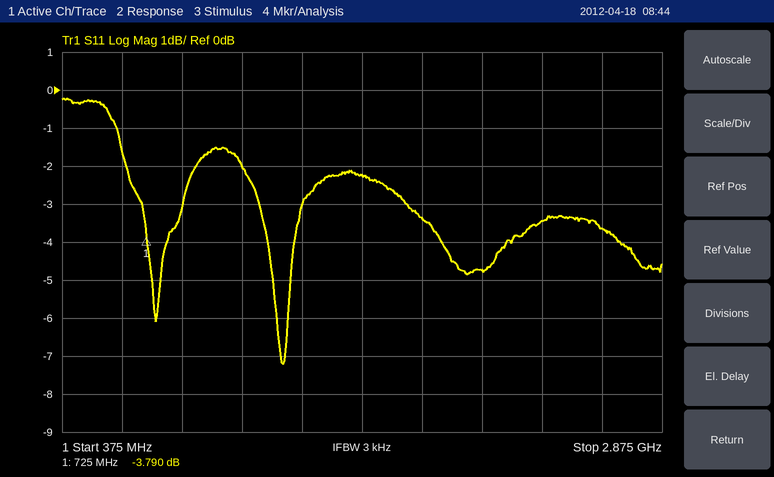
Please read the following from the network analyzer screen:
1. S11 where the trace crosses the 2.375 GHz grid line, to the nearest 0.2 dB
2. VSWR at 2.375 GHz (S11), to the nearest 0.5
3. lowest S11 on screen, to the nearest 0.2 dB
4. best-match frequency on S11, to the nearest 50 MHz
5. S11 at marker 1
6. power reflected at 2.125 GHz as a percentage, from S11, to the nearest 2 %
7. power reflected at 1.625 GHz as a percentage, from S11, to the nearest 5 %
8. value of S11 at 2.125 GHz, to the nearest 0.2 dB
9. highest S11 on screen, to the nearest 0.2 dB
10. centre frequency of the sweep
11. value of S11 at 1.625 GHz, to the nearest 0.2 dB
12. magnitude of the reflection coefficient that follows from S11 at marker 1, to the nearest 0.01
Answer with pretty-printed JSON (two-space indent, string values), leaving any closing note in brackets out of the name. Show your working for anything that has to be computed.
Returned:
{
  "S11 where the trace crosses the 2.375 GHz grid line, to the nearest 0.2 dB": "-3.4 dB",
  "VSWR at 2.375 GHz (S11), to the nearest 0.5": "|Γ| = 10^(-3.4/20) = 0.6761; VSWR = (1 + 0.6761)/(1 − 0.6761) ≈ 5.17, so 5.0 to the nearest 0.5",
  "lowest S11 on screen, to the nearest 0.2 dB": "-7.2 dB",
  "best-match frequency on S11, to the nearest 50 MHz": "1.30 GHz",
  "S11 at marker 1": "-3.790 dB",
  "power reflected at 2.125 GHz as a percentage, from S11, to the nearest 2 %": "10^(-4.8/10) ≈ 33.1 %, so 34 % to the nearest 2 %",
  "power reflected at 1.625 GHz as a percentage, from S11, to the nearest 5 %": "10^(-2.2/10) ≈ 60 %",
  "value of S11 at 2.125 GHz, to the nearest 0.2 dB": "-4.8 dB",
  "highest S11 on screen, to the nearest 0.2 dB": "-0.2 dB",
  "centre frequency of the sweep": "1.625 GHz",
  "value of S11 at 1.625 GHz, to the nearest 0.2 dB": "-2.2 dB",
  "magnitude of the reflection coefficient that follows from S11 at marker 1, to the nearest 0.01": "10^(-3.79/20) ≈ 0.65"
}
